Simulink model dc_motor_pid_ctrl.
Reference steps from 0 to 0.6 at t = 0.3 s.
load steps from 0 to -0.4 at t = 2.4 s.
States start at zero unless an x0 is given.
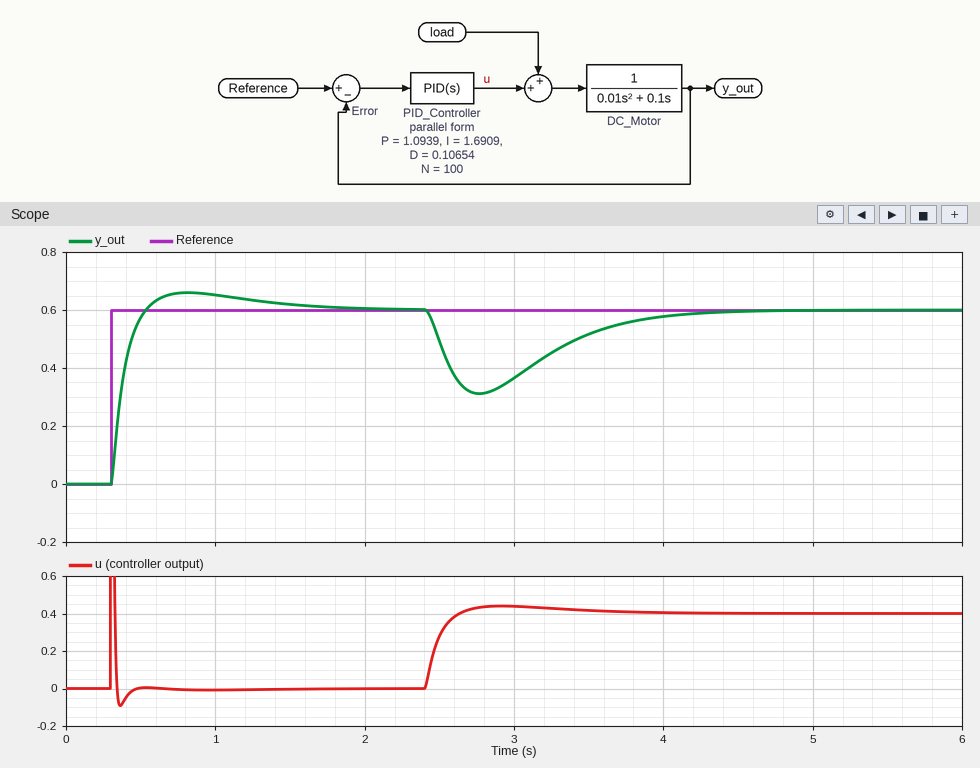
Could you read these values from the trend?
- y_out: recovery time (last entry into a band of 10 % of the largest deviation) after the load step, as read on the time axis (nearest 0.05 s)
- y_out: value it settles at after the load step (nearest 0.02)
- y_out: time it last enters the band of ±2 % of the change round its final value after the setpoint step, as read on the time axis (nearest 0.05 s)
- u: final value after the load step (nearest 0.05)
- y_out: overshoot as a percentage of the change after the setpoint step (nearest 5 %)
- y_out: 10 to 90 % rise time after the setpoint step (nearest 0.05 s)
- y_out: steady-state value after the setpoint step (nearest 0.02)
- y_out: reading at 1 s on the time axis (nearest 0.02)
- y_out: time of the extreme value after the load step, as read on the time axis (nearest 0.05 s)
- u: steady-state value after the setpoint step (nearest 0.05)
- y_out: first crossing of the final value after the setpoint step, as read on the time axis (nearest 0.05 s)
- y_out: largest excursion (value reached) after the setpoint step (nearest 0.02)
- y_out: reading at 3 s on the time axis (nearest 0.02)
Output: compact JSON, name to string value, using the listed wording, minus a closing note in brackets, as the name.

{"y_out: recovery time (last entry into a band of 10 % of the largest deviation) after the load step, as read on the time axis": "3.90 s", "y_out: value it settles at after the load step": "0.60", "y_out: time it last enters the band of ±2 % of the change round its final value after the setpoint step, as read on the time axis": "1.70 s", "u: final value after the load step": "0.40", "y_out: overshoot as a percentage of the change after the setpoint step": "10 %", "y_out: 10 to 90 % rise time after the setpoint step": "0.15 s", "y_out: steady-state value after the setpoint step": "0.60", "y_out: reading at 1 s on the time axis": "0.66", "y_out: time of the extreme value after the load step, as read on the time axis": "2.75 s", "u: steady-state value after the setpoint step": "0.00", "y_out: first crossing of the final value after the setpoint step, as read on the time axis": "0.55 s", "y_out: largest excursion (value reached) after the setpoint step": "0.66", "y_out: reading at 3 s on the time axis": "0.36"}
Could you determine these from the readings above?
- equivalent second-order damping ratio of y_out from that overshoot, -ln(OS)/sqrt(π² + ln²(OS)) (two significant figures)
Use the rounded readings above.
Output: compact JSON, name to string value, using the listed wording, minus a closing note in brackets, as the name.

{"equivalent second-order damping ratio of y_out from that overshoot, -ln(OS)/sqrt(π² + ln²(OS))": "0.59"}
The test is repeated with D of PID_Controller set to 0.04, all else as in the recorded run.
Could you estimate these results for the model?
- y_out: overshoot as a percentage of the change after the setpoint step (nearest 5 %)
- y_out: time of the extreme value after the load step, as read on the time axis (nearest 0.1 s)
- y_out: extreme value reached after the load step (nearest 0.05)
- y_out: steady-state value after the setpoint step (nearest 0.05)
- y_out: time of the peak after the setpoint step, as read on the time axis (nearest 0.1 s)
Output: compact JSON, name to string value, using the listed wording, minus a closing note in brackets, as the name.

{"y_out: overshoot as a percentage of the change after the setpoint step": "20 %", "y_out: time of the extreme value after the load step, as read on the time axis": "2.7 s", "y_out: extreme value reached after the load step": "0.25", "y_out: steady-state value after the setpoint step": "0.60", "y_out: time of the peak after the setpoint step, as read on the time axis": "0.7 s"}
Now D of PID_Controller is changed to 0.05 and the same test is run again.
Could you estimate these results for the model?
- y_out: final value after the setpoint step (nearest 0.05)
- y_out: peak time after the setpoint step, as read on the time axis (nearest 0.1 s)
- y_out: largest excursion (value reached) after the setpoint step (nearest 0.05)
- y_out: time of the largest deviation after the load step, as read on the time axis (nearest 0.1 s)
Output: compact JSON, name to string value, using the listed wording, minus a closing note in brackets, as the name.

{"y_out: final value after the setpoint step": "0.60", "y_out: peak time after the setpoint step, as read on the time axis": "0.7 s", "y_out: largest excursion (value reached) after the setpoint step": "0.70", "y_out: time of the largest deviation after the load step, as read on the time axis": "2.7 s"}
